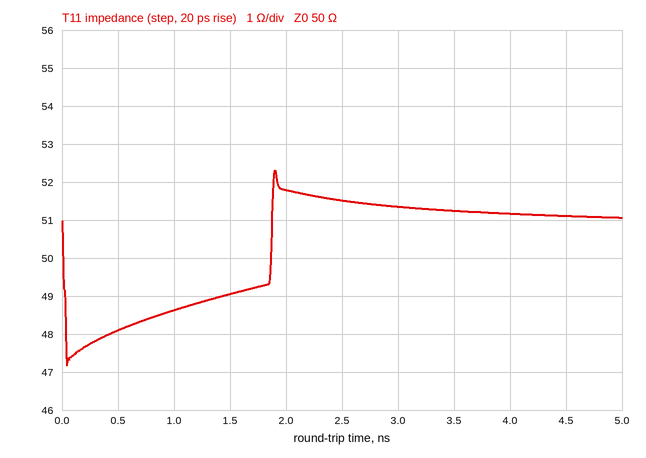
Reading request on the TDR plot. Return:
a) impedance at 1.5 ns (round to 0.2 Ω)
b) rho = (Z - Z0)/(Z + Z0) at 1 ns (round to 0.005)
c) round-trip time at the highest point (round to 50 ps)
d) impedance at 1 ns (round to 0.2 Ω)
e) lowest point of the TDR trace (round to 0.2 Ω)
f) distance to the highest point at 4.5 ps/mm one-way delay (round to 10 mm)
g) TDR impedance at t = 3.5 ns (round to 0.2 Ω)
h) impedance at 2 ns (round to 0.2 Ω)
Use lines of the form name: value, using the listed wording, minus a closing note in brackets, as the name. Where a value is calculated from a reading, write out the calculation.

impedance at 1.5 ns: 49.0 Ω
rho = (Z - Z0)/(Z + Z0) at 1 ns: (48.6 − 50)/(48.6 + 50) ≈ -0.0142, so -0.015 to the nearest 0.005
round-trip time at the highest point: 1.90 ns
impedance at 1 ns: 48.6 Ω
lowest point of the TDR trace: 47.2 Ω
distance to the highest point at 4.5 ps/mm one-way delay: 1.90 ns / 2 / 4.5 ps/mm ≈ 211 mm, so 210 mm to the nearest 10 mm
TDR impedance at t = 3.5 ns: 51.2 Ω
impedance at 2 ns: 51.8 Ω
